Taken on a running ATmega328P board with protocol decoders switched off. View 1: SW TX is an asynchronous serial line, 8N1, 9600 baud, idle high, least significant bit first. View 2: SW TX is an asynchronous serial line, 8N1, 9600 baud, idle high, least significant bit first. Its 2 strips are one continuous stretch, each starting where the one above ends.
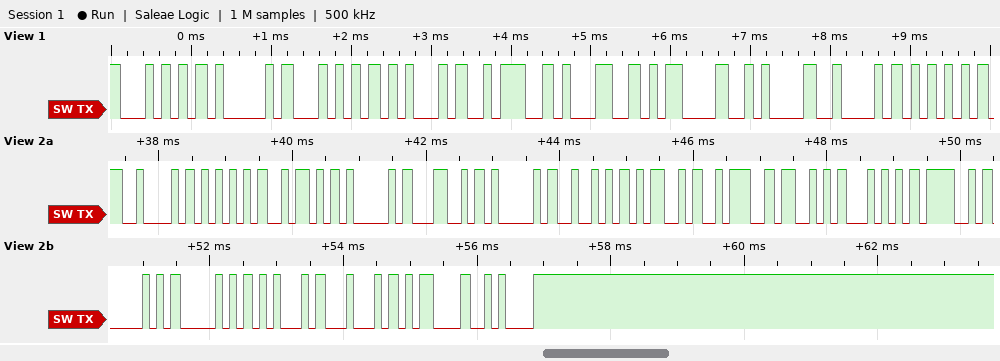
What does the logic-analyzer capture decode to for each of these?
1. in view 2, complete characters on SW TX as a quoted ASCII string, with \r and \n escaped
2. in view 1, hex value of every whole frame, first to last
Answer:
"BUZALARM:STOPPED\r\n"
54 41 54 45 3A 31 0D 0A 42 55
